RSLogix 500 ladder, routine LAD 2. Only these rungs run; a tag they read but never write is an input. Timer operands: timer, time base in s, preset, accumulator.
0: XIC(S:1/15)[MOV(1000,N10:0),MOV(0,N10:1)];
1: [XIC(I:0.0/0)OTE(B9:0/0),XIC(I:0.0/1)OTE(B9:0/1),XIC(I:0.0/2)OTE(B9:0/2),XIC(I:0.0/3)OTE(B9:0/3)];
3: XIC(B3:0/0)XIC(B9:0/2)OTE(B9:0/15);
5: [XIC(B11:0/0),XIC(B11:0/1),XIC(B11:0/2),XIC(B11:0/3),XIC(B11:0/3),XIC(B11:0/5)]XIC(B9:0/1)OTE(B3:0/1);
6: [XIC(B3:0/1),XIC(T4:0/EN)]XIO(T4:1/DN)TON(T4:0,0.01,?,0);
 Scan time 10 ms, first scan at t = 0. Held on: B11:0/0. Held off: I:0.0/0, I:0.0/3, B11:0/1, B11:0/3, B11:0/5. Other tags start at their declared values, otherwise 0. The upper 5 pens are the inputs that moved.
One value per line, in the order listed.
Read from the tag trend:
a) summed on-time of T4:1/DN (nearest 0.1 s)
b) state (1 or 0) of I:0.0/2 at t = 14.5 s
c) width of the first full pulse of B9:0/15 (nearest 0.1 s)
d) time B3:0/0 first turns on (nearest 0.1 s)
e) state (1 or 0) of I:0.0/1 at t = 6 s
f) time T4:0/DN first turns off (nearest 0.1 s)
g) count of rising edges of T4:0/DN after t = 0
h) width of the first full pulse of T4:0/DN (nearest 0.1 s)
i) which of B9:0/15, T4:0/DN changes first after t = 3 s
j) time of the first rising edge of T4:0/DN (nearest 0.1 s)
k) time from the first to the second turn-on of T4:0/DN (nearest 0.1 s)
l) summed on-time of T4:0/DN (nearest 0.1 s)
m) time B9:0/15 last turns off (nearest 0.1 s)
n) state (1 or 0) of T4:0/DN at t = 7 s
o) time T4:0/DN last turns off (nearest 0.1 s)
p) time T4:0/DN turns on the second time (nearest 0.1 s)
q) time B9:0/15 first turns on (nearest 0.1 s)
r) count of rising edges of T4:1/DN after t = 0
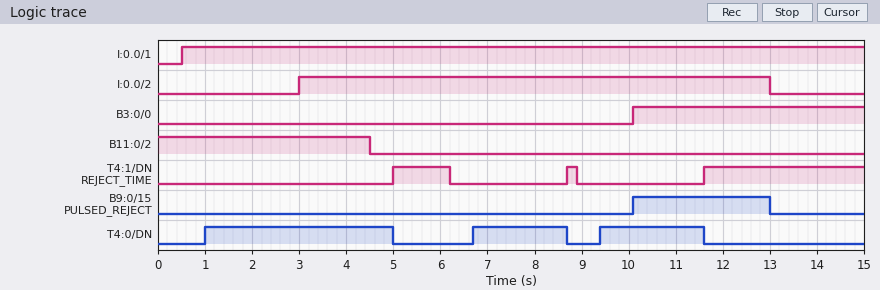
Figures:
4.8 s
0
2.9 s
10.1 s
1
5.0 s
3
4.0 s
T4:0/DN
1.0 s
5.7 s
8.2 s
13.0 s
1
11.6 s
6.7 s
10.1 s
3
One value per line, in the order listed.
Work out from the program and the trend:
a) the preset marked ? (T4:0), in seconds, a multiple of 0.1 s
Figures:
0.5 s
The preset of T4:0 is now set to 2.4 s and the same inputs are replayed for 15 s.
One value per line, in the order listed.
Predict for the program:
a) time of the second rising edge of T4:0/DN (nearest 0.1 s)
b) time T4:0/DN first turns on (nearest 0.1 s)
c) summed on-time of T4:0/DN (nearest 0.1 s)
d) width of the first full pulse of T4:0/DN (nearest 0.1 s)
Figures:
8.6 s
2.9 s
2.5 s
2.1 s
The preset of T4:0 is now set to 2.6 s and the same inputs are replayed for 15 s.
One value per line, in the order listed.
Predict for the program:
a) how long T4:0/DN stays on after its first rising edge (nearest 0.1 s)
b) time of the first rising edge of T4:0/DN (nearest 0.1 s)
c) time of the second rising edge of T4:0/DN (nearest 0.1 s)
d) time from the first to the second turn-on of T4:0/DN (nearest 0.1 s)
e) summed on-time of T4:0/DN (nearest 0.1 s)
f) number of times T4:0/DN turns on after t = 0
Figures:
1.9 s
3.1 s
11.5 s
8.4 s
2.0 s
2
